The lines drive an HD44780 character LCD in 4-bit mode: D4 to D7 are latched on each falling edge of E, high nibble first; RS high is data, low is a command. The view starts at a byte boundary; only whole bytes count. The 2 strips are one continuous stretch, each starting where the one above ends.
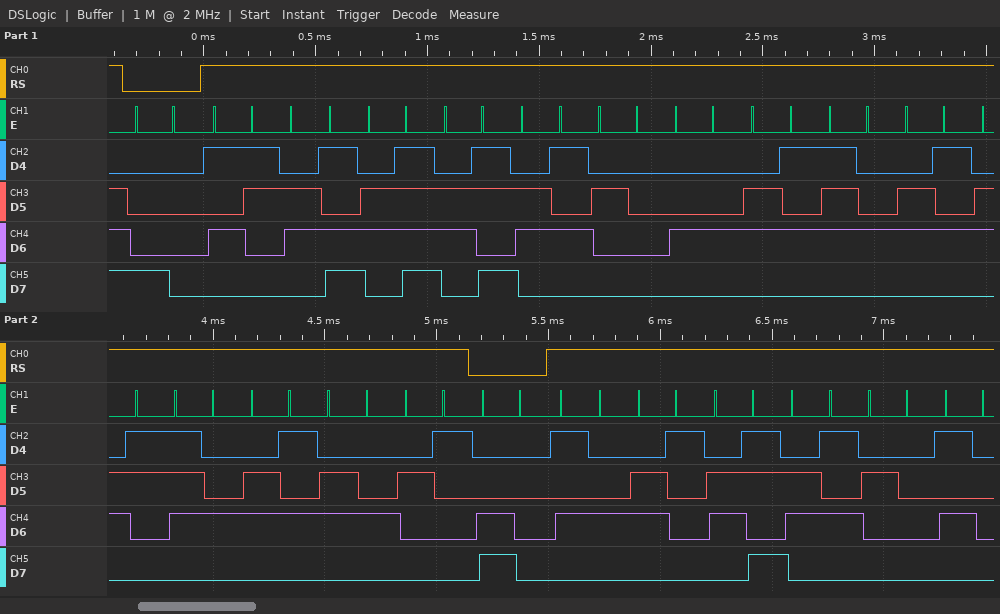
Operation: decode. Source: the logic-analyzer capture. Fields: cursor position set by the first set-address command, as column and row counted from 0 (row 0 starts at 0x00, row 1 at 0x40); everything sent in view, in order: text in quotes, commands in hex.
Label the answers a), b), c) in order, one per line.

a) column 0, row 0
b) 0x80 "Smoke Detected!" 0xC0 "Take P"
